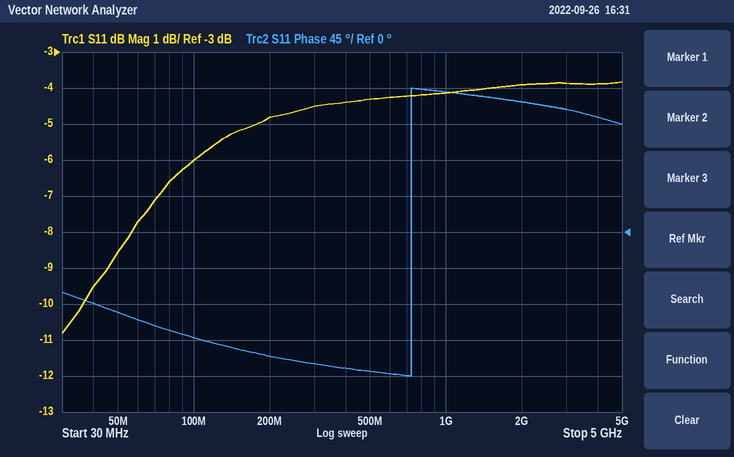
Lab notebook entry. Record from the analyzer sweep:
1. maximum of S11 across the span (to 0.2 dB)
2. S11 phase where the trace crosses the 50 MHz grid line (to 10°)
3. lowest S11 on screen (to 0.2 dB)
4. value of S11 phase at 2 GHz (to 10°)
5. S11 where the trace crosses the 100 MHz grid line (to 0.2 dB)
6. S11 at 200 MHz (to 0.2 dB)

-3.8 dB
-100°
-10.8 dB
160°
-6.0 dB
-4.8 dB
